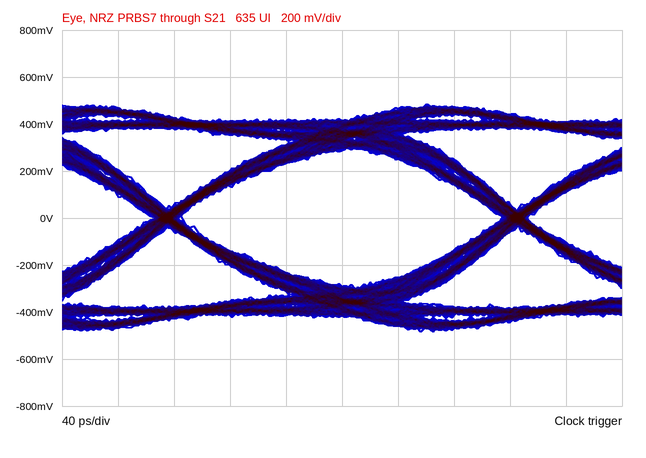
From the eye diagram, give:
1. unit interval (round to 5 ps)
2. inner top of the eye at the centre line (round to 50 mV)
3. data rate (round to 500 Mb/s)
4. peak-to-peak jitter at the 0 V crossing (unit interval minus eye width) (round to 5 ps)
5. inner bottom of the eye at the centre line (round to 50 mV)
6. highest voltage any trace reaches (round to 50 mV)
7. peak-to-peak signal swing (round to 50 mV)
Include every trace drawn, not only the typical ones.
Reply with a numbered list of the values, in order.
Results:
1. 250 ps
2. 300 mV
3. 4.0 Gb/s
4. 20 ps
5. -300 mV
6. 500 mV
7. 950 mV
